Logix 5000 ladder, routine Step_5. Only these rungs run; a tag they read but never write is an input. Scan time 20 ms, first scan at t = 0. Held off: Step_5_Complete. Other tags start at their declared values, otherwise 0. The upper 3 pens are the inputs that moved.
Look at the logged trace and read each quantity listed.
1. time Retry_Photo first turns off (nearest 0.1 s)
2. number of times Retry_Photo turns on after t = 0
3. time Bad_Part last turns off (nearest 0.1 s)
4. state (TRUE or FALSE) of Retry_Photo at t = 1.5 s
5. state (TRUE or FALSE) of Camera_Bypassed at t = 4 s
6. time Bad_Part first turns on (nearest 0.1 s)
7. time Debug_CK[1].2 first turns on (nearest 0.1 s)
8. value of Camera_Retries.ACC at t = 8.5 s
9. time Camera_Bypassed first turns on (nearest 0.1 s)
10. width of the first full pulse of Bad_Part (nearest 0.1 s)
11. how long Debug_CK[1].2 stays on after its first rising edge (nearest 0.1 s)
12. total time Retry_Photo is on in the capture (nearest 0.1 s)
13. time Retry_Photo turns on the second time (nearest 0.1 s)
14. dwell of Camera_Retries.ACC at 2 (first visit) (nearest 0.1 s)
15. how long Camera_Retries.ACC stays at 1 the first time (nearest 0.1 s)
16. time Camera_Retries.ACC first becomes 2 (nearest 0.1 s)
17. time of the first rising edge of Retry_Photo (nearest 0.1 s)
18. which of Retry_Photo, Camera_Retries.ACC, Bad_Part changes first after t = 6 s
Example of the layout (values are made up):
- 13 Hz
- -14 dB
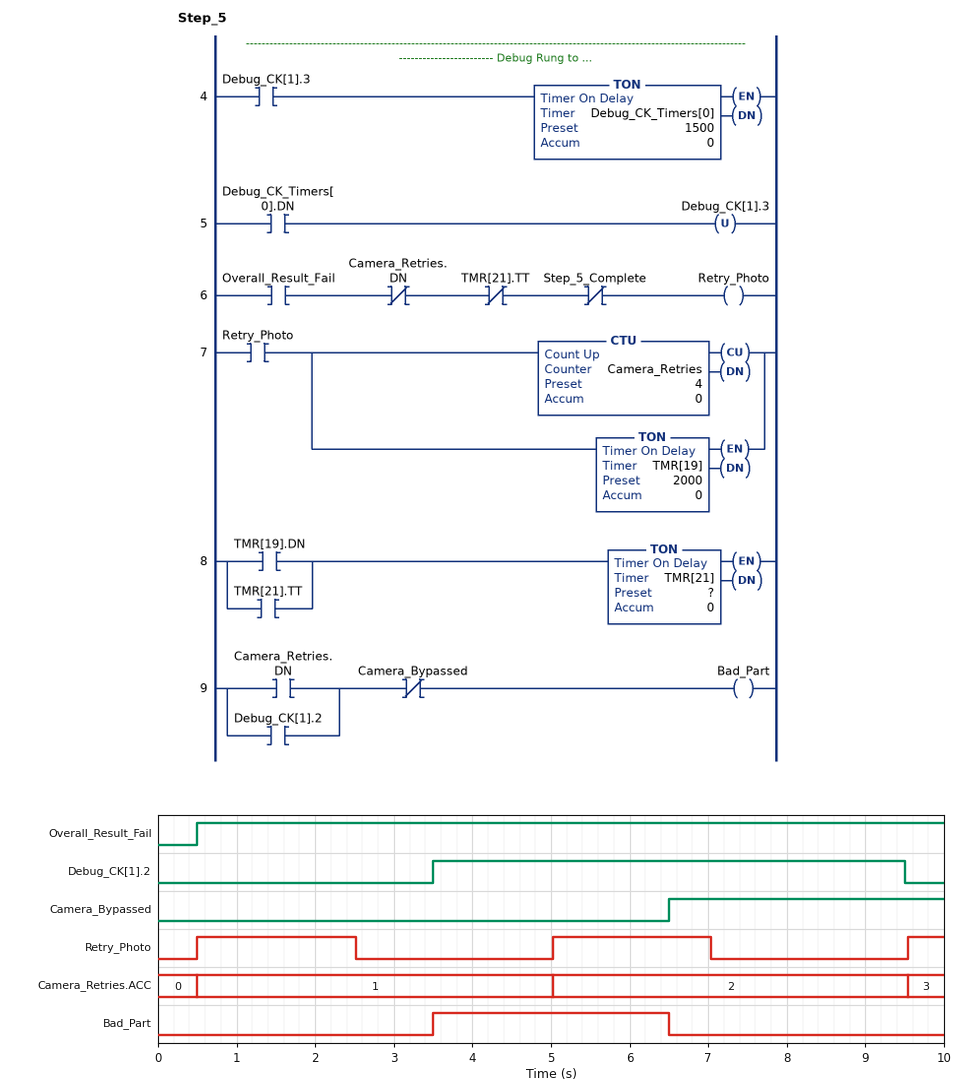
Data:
- 2.5 s
- 3
- 6.5 s
- TRUE
- FALSE
- 3.5 s
- 3.5 s
- 2
- 6.5 s
- 3.0 s
- 6.0 s
- 4.5 s
- 5.0 s
- 4.5 s
- 4.5 s
- 5.0 s
- 0.5 s
- Bad_Part
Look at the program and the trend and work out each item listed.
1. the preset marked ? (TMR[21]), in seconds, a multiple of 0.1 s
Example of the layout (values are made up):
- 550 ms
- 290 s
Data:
- 2.5 s
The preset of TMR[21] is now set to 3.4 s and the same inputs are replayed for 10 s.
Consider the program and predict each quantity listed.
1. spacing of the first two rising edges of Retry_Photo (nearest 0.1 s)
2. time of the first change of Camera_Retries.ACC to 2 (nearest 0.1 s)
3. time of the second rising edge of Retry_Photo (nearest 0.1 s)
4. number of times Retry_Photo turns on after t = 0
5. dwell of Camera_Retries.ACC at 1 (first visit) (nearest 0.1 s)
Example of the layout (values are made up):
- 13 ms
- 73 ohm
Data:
- 5.4 s
- 5.9 s
- 5.9 s
- 2
- 5.4 s
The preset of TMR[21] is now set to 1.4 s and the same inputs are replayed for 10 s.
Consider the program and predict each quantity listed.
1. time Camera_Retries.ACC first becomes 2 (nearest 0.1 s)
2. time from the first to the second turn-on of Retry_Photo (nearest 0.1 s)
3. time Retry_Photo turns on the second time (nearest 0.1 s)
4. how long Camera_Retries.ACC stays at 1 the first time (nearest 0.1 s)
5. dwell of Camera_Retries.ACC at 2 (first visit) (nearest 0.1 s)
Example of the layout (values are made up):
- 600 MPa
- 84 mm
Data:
- 3.9 s
- 3.4 s
- 3.9 s
- 3.4 s
- 3.4 s
